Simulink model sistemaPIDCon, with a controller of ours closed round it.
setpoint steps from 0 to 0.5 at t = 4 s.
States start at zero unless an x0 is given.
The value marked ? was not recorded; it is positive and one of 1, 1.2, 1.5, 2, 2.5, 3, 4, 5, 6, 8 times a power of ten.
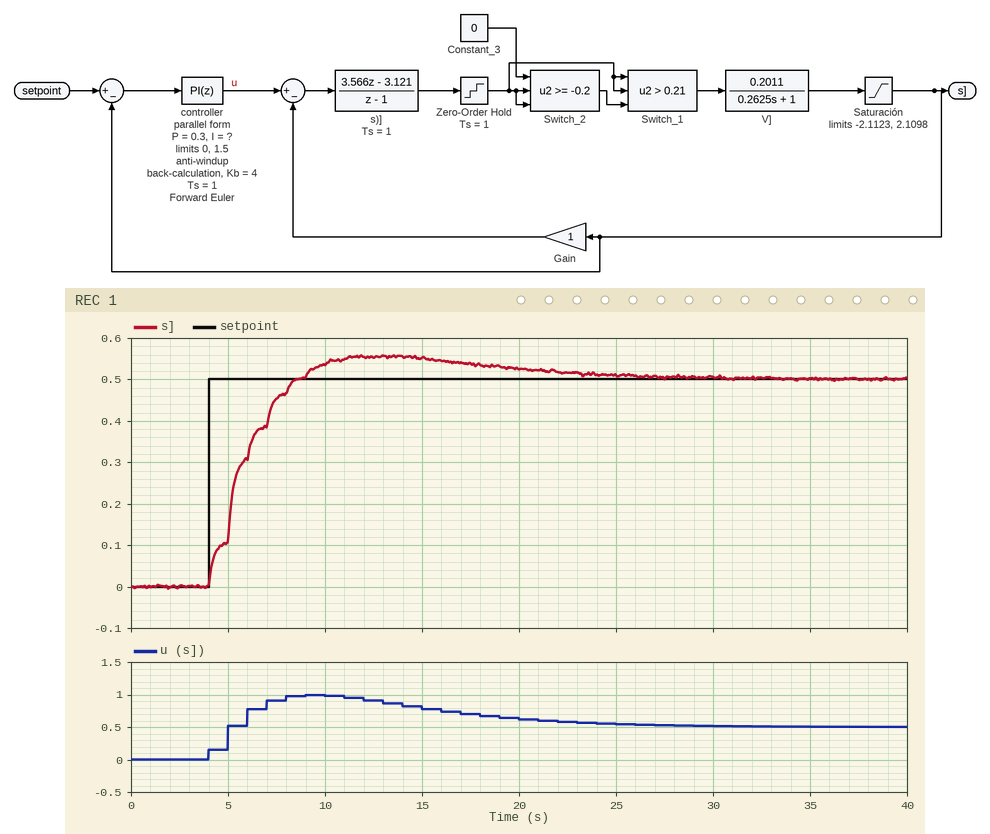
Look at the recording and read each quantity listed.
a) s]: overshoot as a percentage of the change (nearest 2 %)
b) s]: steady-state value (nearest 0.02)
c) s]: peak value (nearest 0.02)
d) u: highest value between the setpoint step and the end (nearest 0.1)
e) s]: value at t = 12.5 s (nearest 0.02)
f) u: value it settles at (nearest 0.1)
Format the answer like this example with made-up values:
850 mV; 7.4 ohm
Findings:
12 %; 0.50; 0.56; 1.0; 0.56; 0.5
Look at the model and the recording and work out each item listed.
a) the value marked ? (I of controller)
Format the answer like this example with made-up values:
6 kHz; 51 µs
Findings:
0.8
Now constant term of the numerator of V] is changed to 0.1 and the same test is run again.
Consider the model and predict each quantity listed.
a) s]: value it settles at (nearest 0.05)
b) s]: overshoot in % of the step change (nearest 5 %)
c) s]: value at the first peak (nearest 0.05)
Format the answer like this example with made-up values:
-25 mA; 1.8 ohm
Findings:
0.50; 20 %; 0.60
